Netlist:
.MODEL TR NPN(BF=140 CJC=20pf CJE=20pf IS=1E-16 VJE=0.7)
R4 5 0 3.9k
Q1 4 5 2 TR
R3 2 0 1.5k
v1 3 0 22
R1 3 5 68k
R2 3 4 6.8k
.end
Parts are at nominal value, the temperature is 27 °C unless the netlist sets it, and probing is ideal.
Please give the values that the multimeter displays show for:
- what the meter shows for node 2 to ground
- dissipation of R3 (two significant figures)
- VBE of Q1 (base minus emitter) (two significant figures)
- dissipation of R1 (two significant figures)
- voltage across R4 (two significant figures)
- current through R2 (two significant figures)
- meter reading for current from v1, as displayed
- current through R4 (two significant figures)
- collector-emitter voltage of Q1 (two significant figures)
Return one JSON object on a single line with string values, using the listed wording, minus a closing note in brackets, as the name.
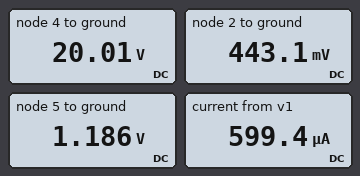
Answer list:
{"what the meter shows for node 2 to ground": "443.1 mV", "dissipation of R3": "130 µW", "VBE of Q1 (base minus emitter)": "740 mV", "dissipation of R1": "6.4 mW", "voltage across R4": "1.2 V", "current through R2": "290 µA", "meter reading for current from v1, as displayed": "599.4 µA", "current through R4": "300 µA", "collector-emitter voltage of Q1": "20 V"}
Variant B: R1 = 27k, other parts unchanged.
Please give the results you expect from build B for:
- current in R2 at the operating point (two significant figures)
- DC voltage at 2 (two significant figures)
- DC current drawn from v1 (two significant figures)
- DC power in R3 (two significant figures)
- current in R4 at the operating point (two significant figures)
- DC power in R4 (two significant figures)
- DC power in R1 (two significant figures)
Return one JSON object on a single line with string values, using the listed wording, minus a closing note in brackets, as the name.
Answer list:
{"current in R2 at the operating point": "1.3 mA", "DC voltage at 2": "2.0 V", "DC current drawn from v1": "2.0 mA", "DC power in R3": "2.6 mW", "current in R4 at the operating point": "700 µA", "DC power in R4": "1.9 mW", "DC power in R1": "14 mW"}
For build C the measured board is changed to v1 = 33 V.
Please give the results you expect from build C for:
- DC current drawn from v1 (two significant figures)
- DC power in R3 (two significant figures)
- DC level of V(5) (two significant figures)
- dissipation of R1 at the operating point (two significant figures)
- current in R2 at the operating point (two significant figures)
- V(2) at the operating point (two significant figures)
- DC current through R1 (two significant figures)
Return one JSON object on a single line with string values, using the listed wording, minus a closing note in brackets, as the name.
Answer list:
{"DC current drawn from v1": "1.1 mA", "DC power in R3": "680 µW", "DC level of V(5)": "1.8 V", "dissipation of R1 at the operating point": "14 mW", "current in R2 at the operating point": "670 µA", "V(2) at the operating point": "1.0 V", "DC current through R1": "460 µA"}
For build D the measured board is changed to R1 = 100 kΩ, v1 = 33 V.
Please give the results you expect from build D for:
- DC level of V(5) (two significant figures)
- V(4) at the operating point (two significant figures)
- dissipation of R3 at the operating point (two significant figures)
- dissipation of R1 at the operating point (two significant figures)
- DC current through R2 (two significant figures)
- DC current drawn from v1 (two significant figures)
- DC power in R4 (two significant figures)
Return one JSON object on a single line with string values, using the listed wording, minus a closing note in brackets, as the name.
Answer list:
{"DC level of V(5)": "1.2 V", "V(4) at the operating point": "31 V", "dissipation of R3 at the operating point": "160 µW", "dissipation of R1 at the operating point": "10 mW", "DC current through R2": "320 µA", "DC current drawn from v1": "640 µA", "DC power in R4": "390 µW"}
